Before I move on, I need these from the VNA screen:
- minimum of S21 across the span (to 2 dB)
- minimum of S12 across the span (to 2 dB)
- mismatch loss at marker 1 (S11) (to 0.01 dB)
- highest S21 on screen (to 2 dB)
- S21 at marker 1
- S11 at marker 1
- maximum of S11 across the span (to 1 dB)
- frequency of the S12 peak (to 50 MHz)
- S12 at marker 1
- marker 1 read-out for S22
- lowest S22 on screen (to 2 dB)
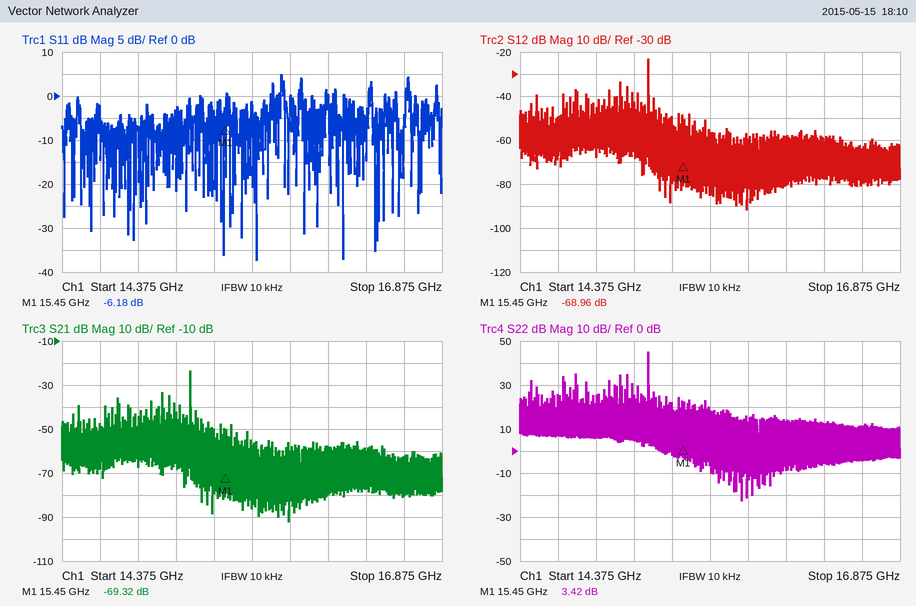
-92 dB
-92 dB
1.20 dB
-24 dB
-69.32 dB
-6.18 dB
5 dB
15.20 GHz
-68.96 dB
3.42 dB
-22 dB
